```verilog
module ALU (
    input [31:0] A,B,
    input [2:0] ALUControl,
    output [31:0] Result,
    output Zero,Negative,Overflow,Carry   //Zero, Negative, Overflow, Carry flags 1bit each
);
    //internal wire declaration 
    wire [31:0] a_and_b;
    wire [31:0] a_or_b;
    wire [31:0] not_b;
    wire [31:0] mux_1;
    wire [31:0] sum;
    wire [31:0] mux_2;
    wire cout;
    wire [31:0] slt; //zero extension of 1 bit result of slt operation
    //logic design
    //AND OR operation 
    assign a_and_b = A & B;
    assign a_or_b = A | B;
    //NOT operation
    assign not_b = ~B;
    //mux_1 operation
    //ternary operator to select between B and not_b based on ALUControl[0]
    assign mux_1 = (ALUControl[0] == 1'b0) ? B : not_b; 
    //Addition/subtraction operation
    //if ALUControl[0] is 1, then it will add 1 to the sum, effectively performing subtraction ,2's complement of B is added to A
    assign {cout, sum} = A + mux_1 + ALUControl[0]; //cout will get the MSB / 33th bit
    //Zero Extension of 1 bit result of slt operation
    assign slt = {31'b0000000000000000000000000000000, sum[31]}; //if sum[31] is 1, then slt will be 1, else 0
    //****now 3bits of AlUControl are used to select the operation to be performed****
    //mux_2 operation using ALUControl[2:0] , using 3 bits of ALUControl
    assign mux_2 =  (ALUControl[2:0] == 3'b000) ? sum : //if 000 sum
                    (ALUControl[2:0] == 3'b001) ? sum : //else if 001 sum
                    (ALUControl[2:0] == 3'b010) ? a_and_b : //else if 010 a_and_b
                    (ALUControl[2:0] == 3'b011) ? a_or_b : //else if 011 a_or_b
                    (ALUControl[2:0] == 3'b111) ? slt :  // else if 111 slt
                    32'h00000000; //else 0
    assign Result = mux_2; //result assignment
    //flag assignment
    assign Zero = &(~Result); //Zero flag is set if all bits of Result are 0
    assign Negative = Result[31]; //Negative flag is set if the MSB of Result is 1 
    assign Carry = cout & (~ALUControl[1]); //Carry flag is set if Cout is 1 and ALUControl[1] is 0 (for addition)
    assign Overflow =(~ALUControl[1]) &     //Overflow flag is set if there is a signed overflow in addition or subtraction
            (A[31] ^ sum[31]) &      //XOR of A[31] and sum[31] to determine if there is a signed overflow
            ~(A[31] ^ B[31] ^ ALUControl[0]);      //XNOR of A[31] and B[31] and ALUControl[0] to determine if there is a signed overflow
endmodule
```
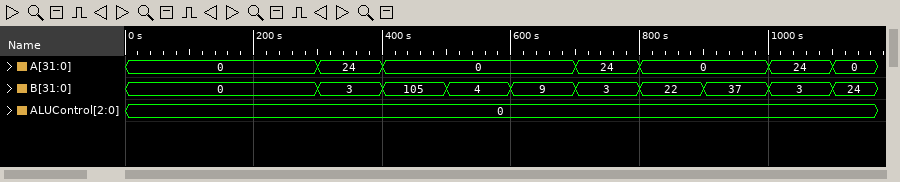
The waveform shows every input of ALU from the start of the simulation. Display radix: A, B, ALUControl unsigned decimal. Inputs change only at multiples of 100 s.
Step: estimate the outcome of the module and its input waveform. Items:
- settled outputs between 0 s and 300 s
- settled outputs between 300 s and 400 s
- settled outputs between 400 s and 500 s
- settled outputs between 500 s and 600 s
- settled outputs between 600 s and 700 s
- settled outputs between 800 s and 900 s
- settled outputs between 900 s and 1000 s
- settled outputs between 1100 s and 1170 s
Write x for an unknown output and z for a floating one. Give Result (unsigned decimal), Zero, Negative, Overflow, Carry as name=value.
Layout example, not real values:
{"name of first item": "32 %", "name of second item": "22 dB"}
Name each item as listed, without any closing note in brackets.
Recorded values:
{"settled outputs between 0 s and 300 s": "Result=0, Zero=1, Negative=0, Overflow=0, Carry=0", "settled outputs between 300 s and 400 s": "Result=27, Zero=0, Negative=0, Overflow=0, Carry=0", "settled outputs between 400 s and 500 s": "Result=105, Zero=0, Negative=0, Overflow=0, Carry=0", "settled outputs between 500 s and 600 s": "Result=4, Zero=0, Negative=0, Overflow=0, Carry=0", "settled outputs between 600 s and 700 s": "Result=9, Zero=0, Negative=0, Overflow=0, Carry=0", "settled outputs between 800 s and 900 s": "Result=22, Zero=0, Negative=0, Overflow=0, Carry=0", "settled outputs between 900 s and 1000 s": "Result=37, Zero=0, Negative=0, Overflow=0, Carry=0", "settled outputs between 1100 s and 1170 s": "Result=24, Zero=0, Negative=0, Overflow=0, Carry=0"}
